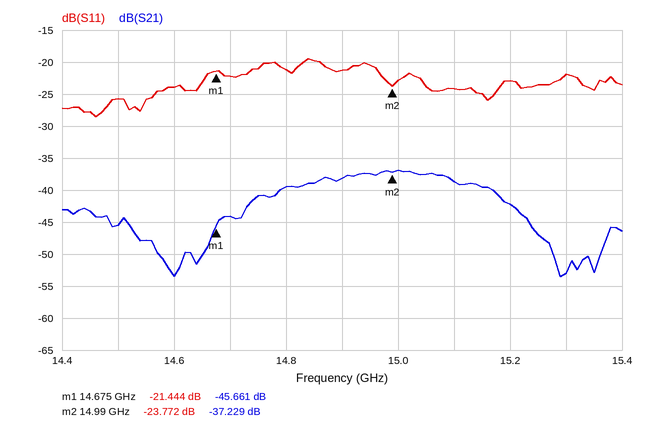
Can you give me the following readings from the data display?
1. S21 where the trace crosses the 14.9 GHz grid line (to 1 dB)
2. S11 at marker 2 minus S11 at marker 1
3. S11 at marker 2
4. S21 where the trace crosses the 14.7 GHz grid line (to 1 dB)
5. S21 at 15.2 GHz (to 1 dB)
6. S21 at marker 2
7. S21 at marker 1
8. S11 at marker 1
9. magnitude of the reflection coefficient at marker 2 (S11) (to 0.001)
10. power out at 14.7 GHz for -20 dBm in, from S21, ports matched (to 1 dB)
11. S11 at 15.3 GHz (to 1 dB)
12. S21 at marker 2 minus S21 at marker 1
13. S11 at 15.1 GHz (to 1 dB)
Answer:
-38 dB
-2.328 dB
-23.772 dB
-44 dB
-42 dB
-37.229 dB
-45.661 dB
-21.444 dB
0.065
-64 dBm
-22 dB
8.432 dB
-24 dB
